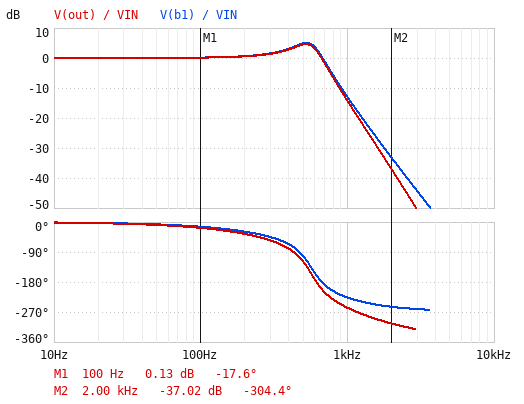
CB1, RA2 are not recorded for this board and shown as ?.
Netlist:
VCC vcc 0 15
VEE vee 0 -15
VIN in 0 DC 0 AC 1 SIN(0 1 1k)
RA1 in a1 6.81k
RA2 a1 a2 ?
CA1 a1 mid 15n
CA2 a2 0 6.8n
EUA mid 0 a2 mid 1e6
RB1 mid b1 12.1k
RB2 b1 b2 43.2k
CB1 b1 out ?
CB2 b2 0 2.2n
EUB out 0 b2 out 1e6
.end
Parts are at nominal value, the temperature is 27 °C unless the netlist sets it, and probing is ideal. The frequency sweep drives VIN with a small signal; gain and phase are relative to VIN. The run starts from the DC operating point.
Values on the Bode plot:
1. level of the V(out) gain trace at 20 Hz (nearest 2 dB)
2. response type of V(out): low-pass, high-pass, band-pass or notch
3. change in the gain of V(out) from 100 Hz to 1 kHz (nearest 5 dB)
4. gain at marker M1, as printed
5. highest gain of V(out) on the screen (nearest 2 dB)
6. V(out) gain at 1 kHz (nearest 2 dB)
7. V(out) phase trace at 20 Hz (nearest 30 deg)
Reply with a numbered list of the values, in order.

1. 0 dB
2. low-pass
3. -15 dB
4. 0.13 dB
5. 4 dB
6. -14 dB
7. 0 deg
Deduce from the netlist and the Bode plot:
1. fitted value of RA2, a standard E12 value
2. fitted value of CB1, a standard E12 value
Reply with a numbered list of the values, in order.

1. 47 kΩ
2. 68 nF
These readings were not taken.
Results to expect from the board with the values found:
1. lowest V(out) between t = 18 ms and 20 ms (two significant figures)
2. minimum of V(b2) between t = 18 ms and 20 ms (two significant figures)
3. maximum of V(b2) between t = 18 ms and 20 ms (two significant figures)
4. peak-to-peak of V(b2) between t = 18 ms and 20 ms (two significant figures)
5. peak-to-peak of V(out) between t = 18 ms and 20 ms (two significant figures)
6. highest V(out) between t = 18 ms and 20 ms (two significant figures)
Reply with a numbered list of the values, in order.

1. -190 mV
2. -190 mV
3. 190 mV
4. 390 mV
5. 390 mV
6. 190 mV
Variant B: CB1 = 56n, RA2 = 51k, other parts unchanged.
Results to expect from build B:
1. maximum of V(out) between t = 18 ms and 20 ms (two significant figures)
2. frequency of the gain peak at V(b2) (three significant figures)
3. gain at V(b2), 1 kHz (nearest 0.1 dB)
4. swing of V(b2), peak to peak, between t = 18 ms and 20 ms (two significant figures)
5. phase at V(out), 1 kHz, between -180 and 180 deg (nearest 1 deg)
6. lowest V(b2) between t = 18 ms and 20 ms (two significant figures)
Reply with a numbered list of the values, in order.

1. 230 mV
2. 559 Hz
3. -12.7 dB
4. 460 mV
5. 107 deg
6. -230 mV
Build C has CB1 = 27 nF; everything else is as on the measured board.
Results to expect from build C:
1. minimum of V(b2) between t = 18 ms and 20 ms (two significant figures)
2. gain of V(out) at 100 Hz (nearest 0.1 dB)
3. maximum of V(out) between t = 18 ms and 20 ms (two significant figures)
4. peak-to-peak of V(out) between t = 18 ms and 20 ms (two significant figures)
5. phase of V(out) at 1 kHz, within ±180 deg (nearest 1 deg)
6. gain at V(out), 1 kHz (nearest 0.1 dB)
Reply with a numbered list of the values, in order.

1. -540 mV
2. 0 dB
3. 540 mV
4. 1.1 V
5. 156 deg
6. -5.3 dB
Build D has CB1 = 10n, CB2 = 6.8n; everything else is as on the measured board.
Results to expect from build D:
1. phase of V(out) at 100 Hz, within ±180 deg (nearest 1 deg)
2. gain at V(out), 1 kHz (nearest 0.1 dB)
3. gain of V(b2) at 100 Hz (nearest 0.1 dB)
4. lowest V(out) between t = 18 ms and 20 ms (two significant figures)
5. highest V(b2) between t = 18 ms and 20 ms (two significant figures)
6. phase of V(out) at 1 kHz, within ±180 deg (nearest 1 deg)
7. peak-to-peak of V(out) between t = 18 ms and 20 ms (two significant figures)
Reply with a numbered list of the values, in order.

1. -27 deg
2. -14.9 dB
3. -0.2 dB
4. -180 mV
5. 180 mV
6. 163 deg
7. 360 mV
